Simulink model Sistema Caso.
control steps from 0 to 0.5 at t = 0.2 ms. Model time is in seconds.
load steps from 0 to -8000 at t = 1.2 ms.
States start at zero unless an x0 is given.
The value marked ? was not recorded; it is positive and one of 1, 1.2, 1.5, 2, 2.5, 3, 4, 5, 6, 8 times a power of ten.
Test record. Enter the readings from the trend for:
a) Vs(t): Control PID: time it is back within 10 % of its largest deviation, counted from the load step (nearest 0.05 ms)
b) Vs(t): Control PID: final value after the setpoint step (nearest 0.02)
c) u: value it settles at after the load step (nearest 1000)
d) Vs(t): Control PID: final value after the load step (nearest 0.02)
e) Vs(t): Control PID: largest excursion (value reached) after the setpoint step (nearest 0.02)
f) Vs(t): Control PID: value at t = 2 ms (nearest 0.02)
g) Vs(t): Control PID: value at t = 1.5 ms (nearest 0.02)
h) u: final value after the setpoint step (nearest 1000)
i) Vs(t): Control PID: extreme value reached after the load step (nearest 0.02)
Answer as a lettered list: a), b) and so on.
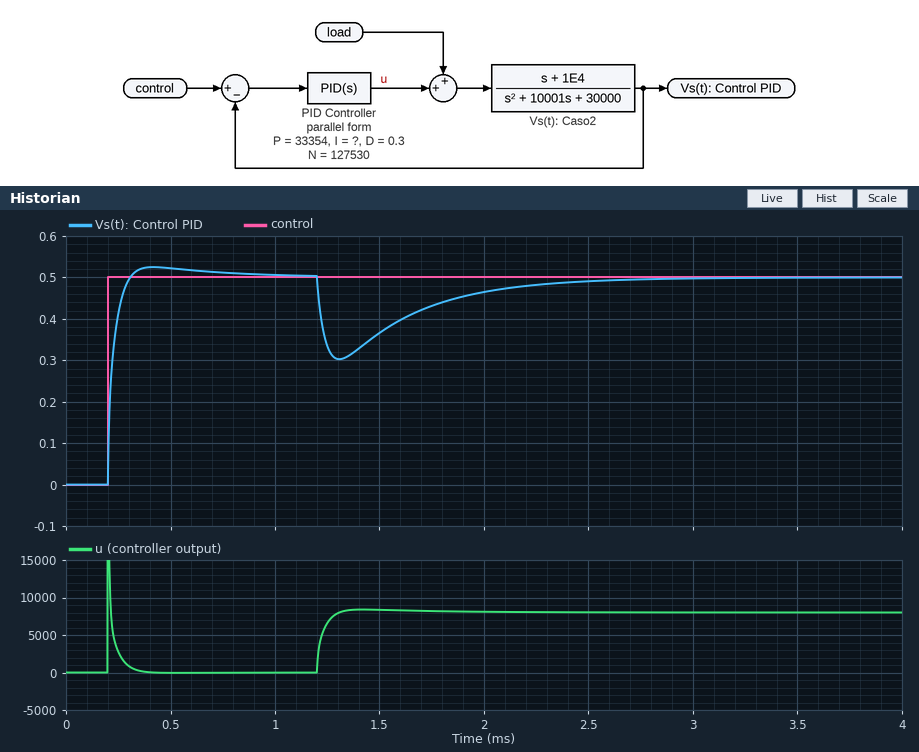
a) 1.00 ms
b) 0.50
c) 8000
d) 0.50
e) 0.52
f) 0.46
g) 0.36
h) 0
i) 0.30
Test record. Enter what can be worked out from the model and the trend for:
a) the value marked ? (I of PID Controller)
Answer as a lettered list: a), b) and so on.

a) 8e+07
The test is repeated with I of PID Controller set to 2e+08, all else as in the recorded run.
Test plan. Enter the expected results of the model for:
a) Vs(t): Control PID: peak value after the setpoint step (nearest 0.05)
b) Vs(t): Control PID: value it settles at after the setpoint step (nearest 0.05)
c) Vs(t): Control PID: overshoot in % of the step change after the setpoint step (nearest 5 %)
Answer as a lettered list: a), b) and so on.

a) 0.55
b) 0.50
c) 10 %
